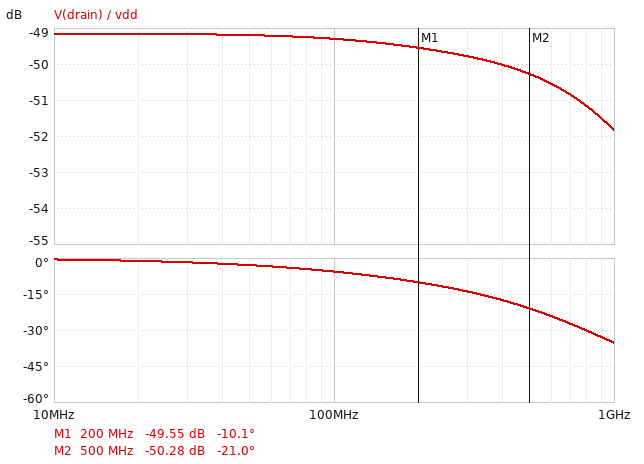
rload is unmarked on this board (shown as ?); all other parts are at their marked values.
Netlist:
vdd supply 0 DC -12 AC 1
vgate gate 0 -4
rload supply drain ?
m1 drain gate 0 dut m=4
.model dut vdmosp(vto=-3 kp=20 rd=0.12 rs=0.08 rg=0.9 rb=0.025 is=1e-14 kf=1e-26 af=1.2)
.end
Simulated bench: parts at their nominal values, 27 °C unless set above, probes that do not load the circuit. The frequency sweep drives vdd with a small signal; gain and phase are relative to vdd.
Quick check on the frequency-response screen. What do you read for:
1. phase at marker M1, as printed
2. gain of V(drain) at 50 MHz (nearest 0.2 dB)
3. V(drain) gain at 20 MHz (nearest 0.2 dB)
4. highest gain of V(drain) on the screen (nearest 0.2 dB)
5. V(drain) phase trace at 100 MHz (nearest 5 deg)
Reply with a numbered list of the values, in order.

1. -10.1 deg
2. -49.2 dB
3. -49.2 dB
4. -49.2 dB
5. -5 deg
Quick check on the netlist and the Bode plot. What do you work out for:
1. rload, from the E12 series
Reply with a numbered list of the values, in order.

1. 18 Ω
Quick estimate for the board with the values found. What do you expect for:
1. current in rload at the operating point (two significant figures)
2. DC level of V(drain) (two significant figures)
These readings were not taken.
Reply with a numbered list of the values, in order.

1. 660 mA
2. -42 mV
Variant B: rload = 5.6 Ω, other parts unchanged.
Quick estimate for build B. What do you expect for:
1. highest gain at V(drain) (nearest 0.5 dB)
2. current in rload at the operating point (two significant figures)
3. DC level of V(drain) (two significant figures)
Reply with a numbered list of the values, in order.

1. -39.0 dB
2. 2.1 A
3. -130 mV
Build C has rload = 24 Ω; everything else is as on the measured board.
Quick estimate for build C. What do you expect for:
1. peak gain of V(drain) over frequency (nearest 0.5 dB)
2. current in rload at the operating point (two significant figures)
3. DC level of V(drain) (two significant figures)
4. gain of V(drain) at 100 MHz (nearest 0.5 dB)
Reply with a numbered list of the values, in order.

1. -51.5 dB
2. 500 mA
3. -31 mV
4. -52.0 dB
